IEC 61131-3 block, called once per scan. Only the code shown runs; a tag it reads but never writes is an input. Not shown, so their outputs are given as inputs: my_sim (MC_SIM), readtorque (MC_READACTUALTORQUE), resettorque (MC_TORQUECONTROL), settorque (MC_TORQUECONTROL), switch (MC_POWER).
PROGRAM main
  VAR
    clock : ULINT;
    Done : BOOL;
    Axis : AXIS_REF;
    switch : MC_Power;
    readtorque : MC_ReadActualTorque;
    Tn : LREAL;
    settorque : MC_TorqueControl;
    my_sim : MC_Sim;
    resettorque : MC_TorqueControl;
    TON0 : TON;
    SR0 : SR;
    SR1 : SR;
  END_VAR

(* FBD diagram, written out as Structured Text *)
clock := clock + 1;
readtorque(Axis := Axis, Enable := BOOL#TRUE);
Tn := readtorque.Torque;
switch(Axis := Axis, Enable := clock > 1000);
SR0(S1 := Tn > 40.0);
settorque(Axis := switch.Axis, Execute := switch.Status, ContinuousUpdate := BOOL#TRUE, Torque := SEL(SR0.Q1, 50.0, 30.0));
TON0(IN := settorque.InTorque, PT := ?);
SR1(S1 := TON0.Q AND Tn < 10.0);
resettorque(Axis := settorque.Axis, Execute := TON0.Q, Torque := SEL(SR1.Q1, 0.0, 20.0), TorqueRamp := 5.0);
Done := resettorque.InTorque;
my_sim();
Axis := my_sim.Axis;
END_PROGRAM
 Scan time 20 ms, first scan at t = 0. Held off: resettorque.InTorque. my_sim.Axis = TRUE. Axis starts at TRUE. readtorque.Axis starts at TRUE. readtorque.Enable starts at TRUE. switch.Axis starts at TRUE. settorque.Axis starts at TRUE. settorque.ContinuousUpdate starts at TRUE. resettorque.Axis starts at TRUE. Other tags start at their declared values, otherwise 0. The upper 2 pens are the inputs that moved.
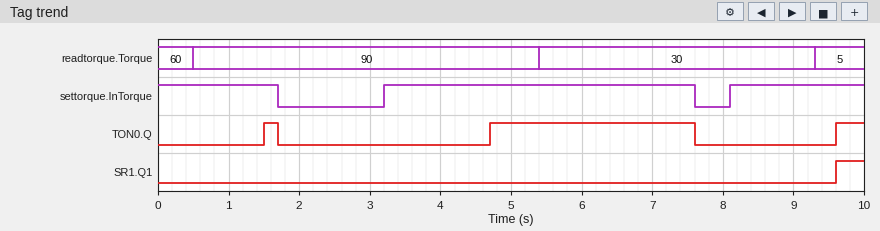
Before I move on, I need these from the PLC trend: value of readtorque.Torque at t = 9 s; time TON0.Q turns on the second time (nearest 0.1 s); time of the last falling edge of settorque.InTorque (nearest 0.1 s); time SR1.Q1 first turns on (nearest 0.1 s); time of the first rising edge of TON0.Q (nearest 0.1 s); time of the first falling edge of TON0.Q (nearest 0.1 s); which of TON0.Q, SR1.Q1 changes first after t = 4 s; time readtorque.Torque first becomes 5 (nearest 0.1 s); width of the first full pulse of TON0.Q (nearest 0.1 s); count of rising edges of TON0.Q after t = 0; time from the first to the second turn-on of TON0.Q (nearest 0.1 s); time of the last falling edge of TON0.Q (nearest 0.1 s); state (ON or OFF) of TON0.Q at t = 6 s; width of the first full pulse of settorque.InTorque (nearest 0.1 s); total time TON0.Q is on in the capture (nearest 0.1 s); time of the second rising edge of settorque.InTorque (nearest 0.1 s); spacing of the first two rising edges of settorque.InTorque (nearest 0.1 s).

30
4.7 s
7.6 s
9.6 s
1.5 s
1.7 s
TON0.Q
9.3 s
0.2 s
3
3.2 s
7.6 s
ON
4.4 s
3.5 s
8.1 s
4.9 s
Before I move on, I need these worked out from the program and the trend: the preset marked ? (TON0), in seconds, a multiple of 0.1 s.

1.5 s
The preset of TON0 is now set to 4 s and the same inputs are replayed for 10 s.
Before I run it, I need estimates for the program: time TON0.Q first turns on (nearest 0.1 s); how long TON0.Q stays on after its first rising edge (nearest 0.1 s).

7.2 s
0.4 s
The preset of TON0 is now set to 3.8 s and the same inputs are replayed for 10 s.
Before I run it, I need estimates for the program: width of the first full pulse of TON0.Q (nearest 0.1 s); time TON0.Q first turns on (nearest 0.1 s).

0.6 s
7.0 s
